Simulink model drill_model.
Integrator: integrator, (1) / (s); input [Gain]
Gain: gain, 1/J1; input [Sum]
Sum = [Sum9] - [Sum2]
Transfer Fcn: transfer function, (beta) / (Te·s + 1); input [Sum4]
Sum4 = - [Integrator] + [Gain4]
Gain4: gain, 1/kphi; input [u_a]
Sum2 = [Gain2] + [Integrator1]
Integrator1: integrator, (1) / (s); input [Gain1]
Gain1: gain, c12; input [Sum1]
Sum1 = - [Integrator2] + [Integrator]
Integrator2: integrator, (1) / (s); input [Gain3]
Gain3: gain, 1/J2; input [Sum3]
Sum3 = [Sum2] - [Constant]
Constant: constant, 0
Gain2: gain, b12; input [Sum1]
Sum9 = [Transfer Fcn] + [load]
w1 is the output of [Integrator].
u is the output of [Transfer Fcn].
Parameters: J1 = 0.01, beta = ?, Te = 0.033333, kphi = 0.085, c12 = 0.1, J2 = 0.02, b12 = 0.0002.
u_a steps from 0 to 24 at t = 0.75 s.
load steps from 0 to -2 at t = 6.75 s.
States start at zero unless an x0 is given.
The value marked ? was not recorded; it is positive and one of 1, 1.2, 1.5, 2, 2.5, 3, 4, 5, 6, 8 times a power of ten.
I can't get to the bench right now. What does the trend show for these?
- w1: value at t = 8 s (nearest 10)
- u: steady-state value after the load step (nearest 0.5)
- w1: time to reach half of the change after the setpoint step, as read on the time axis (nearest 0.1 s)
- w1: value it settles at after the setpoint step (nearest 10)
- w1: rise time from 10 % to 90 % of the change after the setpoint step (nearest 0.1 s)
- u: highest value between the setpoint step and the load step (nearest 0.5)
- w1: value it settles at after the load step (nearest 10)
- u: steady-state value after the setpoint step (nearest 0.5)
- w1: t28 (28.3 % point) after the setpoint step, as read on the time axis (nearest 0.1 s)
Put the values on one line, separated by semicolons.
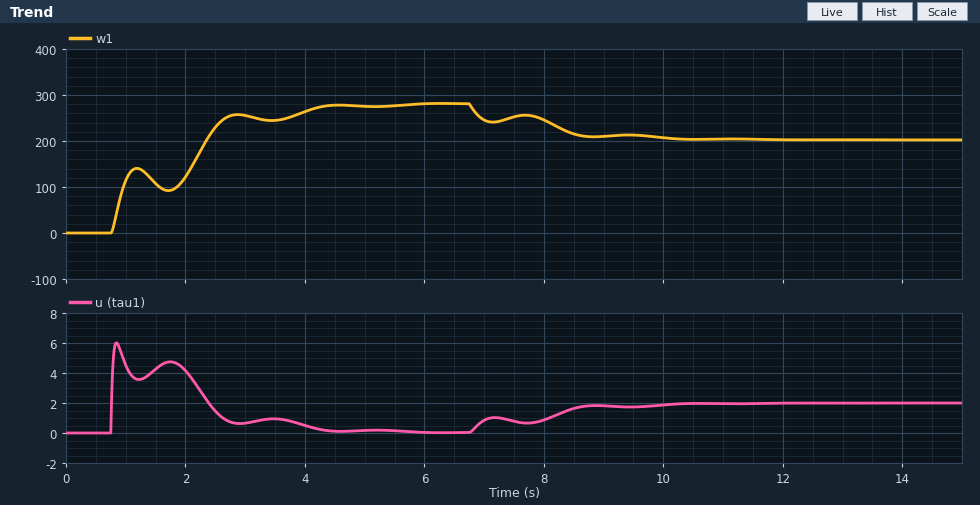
250; 2.0; 2.1 s; 280; 1.9 s; 6.0; 200; 0.0; 0.9 s
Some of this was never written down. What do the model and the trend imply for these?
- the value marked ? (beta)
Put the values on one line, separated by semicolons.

0.025
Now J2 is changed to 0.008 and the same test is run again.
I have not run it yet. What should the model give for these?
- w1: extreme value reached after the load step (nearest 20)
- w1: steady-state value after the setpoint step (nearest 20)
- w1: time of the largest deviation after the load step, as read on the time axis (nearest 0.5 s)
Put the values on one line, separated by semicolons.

200; 280; 9.5 s
